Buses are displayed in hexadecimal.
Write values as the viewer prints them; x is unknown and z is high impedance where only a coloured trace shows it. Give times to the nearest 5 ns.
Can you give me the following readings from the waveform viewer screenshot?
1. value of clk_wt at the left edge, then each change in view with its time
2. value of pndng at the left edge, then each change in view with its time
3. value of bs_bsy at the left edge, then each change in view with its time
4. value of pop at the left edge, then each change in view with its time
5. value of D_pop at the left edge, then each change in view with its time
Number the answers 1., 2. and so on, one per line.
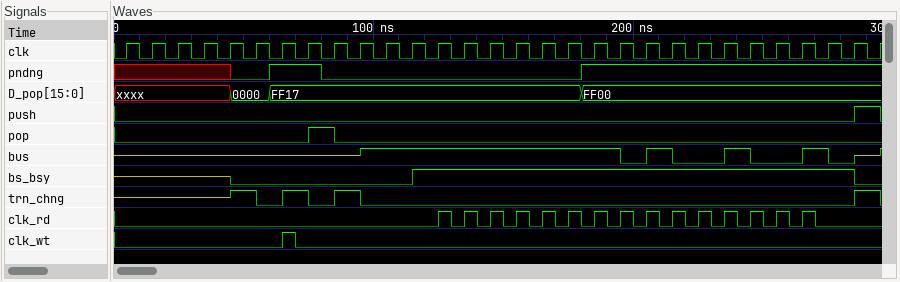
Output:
1. 0, 1 at 65 ns, 0 at 70 ns
2. x, 0 at 45 ns, 1 at 60 ns, 0 at 80 ns, 1 at 180 ns
3. z, 0 at 45 ns, 1 at 115 ns, 0 at 285 ns
4. 0, 1 at 75 ns, 0 at 85 ns
5. xxxx, 0000 at 45 ns, FF17 at 60 ns, FF00 at 180 ns
